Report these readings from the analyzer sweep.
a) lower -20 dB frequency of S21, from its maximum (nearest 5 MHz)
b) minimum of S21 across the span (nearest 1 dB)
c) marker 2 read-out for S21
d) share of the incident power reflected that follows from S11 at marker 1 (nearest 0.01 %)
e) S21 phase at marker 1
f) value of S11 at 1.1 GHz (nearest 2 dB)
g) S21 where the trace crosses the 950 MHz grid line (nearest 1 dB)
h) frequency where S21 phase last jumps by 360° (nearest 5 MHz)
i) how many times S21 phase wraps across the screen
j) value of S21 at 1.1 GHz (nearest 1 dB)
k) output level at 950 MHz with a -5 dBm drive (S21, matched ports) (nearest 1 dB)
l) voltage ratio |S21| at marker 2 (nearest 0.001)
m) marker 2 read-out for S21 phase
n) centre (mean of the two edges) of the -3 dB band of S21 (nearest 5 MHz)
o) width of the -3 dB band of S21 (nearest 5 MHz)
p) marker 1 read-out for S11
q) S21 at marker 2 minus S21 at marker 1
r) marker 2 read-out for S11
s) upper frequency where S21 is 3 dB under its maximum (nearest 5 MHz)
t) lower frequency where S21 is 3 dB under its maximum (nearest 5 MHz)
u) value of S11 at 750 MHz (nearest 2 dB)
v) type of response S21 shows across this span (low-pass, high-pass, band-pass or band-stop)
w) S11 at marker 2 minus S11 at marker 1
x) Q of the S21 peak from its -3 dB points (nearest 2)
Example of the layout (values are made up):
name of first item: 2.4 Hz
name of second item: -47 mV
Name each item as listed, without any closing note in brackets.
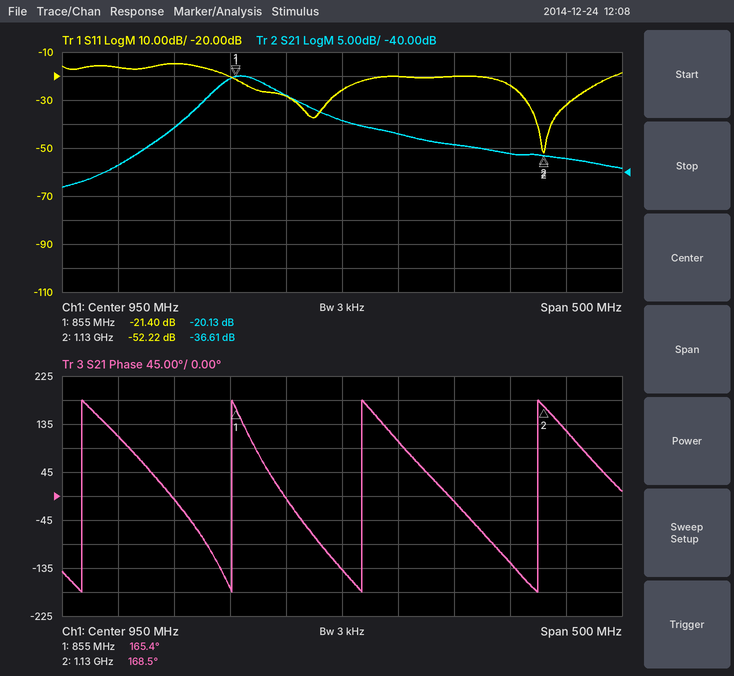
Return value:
lower -20 dB frequency of S21, from its maximum: 740 MHz
minimum of S21 across the span: -43 dB
marker 2 read-out for S21: -36.61 dB
share of the incident power reflected that follows from S11 at marker 1: 0.72 %
S21 phase at marker 1: 165.4°
value of S11 at 1.1 GHz: -24 dB
S21 where the trace crosses the 950 MHz grid line: -29 dB
frequency where S21 phase last jumps by 360°: 1.125 GHz
how many times S21 phase wraps across the screen: 4
value of S21 at 1.1 GHz: -36 dB
output level at 950 MHz with a -5 dBm drive (S21, matched ports): -34 dBm
voltage ratio |S21| at marker 2: 0.015
marker 2 read-out for S21 phase: 168.5°
centre (mean of the two edges) of the -3 dB band of S21: 865 MHz
width of the -3 dB band of S21: 55 MHz
marker 1 read-out for S11: -21.40 dB
S21 at marker 2 minus S21 at marker 1: -16.48 dB
marker 2 read-out for S11: -52.22 dB
upper frequency where S21 is 3 dB under its maximum: 890 MHz
lower frequency where S21 is 3 dB under its maximum: 835 MHz
value of S11 at 750 MHz: -16 dB
type of response S21 shows across this span: band-pass
S11 at marker 2 minus S11 at marker 1: -30.82 dB
Q of the S21 peak from its -3 dB points: 16
